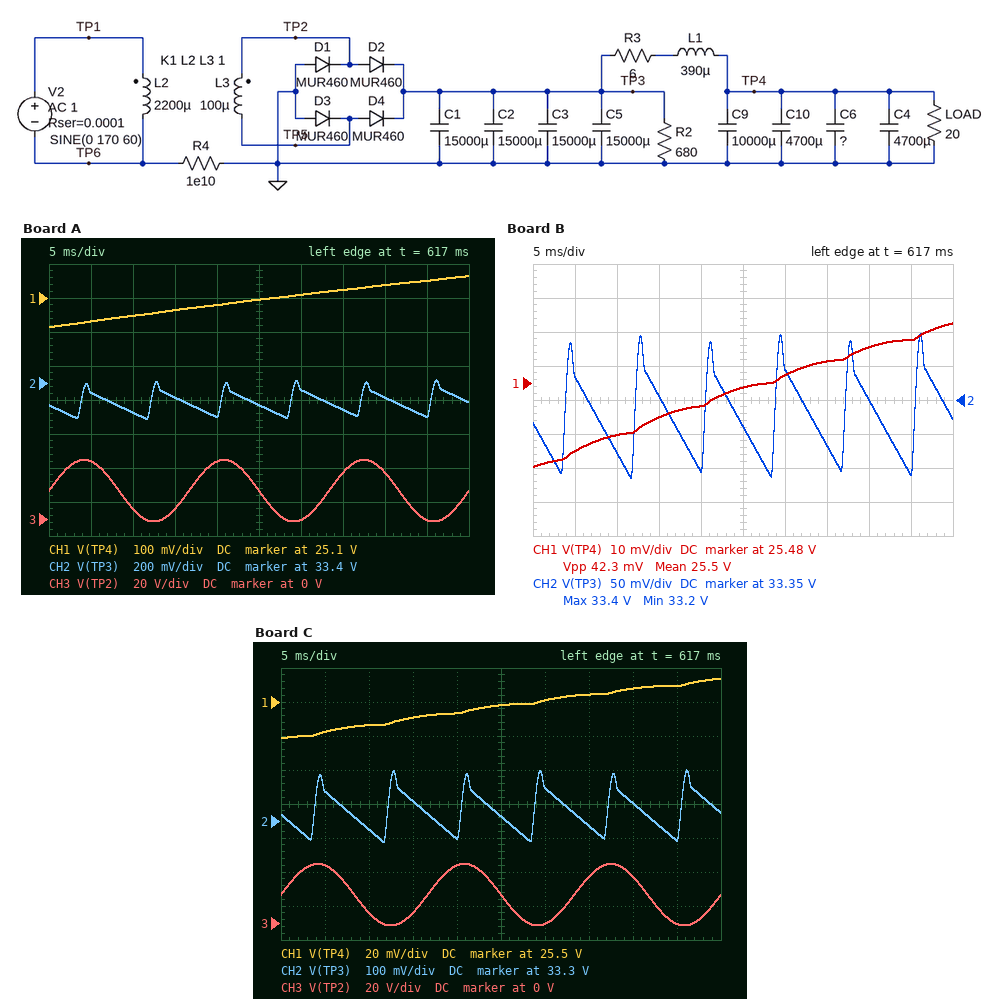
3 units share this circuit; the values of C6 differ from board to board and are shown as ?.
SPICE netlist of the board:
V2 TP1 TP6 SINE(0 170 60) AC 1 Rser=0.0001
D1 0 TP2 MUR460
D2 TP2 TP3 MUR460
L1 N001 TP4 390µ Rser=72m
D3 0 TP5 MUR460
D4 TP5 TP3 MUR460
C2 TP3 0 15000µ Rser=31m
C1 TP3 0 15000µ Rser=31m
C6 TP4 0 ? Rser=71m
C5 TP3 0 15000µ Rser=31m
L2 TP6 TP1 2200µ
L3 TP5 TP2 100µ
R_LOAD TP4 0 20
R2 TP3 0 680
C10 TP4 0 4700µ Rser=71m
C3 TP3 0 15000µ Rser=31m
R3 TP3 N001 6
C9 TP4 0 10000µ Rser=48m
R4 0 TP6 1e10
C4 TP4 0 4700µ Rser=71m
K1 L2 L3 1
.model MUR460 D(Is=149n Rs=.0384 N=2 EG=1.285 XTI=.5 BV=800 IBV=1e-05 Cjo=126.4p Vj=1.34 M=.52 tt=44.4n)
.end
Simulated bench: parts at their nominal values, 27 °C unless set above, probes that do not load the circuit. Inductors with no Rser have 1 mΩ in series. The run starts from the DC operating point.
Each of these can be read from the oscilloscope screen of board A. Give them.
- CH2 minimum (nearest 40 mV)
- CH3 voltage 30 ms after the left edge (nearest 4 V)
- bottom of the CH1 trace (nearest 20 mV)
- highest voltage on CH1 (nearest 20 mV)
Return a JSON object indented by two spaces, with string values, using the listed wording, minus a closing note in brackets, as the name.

{
  "CH2 minimum": "33.20 V",
  "CH3 voltage 30 ms after the left edge": "0 V",
  "bottom of the CH1 trace": "25.02 V",
  "highest voltage on CH1": "25.16 V"
}
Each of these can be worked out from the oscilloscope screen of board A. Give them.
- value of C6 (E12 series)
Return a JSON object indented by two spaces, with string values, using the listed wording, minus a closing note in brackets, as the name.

{
  "value of C6": "12 mF"
}
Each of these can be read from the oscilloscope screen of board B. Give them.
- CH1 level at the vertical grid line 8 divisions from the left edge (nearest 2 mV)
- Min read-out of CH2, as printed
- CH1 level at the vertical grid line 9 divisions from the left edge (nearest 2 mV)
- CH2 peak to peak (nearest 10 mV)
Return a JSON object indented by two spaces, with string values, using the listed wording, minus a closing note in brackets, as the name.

{
  "CH1 level at the vertical grid line 8 divisions from the left edge": "25.490 V",
  "Min read-out of CH2, as printed": "33.2 V",
  "CH1 level at the vertical grid line 9 divisions from the left edge": "25.492 V",
  "CH2 peak to peak": "210 mV"
}
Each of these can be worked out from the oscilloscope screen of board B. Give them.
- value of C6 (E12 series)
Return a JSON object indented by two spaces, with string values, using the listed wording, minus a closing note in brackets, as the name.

{
  "value of C6": "2.7 mF"
}
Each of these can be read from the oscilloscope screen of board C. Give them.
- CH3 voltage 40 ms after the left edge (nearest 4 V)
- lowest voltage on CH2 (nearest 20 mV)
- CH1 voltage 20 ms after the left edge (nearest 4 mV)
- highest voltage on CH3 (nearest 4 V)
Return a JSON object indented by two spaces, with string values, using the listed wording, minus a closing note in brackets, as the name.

{
  "CH3 voltage 40 ms after the left edge": "28 V",
  "lowest voltage on CH2": "33.24 V",
  "CH1 voltage 20 ms after the left edge": "25.492 V",
  "highest voltage on CH3": "36 V"
}
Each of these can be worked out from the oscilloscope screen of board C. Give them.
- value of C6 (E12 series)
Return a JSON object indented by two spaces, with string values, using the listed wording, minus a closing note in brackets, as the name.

{
  "value of C6": "1.8 mF"
}
